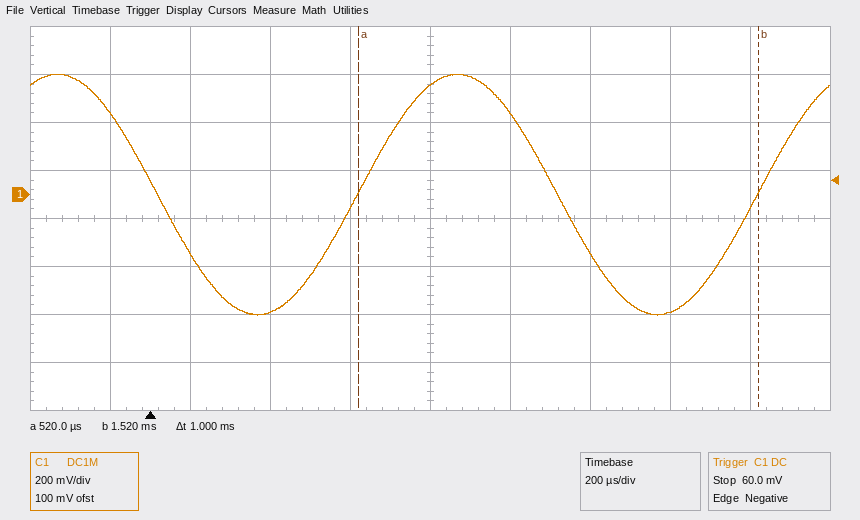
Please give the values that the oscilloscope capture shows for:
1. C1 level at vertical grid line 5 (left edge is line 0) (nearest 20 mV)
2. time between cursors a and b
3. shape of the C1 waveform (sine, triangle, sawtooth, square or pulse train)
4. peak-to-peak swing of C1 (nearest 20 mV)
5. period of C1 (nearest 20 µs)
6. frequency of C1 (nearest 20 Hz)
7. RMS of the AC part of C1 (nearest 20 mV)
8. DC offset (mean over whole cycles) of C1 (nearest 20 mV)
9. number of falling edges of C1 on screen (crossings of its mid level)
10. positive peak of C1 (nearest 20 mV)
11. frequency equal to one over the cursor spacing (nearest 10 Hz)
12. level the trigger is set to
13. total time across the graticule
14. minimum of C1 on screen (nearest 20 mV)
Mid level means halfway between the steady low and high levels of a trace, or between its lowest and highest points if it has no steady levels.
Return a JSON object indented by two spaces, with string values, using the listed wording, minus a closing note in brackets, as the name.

{
  "C1 level at vertical grid line 5 (left edge is line 0)": "460 mV",
  "time between cursors a and b": "1 ms",
  "shape of the C1 waveform": "sine",
  "peak-to-peak swing of C1": "1.00 V",
  "period of C1": "1.00 ms",
  "frequency of C1": "1.00 kHz",
  "RMS of the AC part of C1": "360 mV",
  "DC offset (mean over whole cycles) of C1": "0 mV",
  "number of falling edges of C1 on screen": "2",
  "positive peak of C1": "500 mV",
  "frequency equal to one over the cursor spacing": "1.00 kHz",
  "level the trigger is set to": "60.0 mV",
  "total time across the graticule": "2 ms",
  "minimum of C1 on screen": "-500 mV"
}
